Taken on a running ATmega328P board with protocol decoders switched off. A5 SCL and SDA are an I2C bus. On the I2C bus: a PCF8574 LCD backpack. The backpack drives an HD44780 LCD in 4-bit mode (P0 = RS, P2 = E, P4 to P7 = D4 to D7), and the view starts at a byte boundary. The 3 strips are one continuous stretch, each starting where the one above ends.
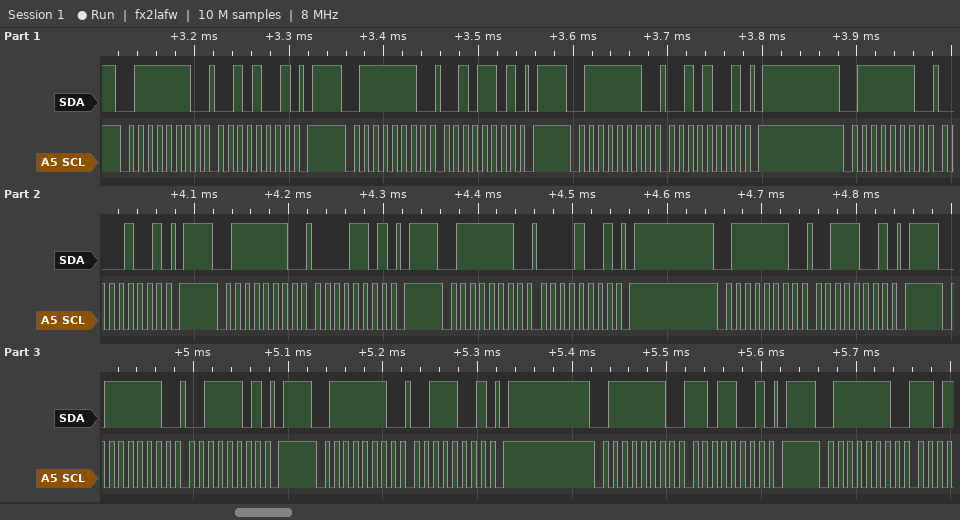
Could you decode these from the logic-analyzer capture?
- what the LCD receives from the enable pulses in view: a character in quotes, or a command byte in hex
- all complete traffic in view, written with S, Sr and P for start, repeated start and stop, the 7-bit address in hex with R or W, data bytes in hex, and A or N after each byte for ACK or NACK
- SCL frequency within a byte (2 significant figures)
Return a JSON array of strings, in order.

["' '", "S 3FW A 29 A P S 3FW A 2D A P S 3FW A 29 A P S 3FW A 09 A P S 3FW A 0D A P S 3FW A 09 A P S 3FW A 39 A P S 3FW A 3D A P S 3FW A 39 A P S 3FW A D9 A P S 3FW A", "100 kHz"]
